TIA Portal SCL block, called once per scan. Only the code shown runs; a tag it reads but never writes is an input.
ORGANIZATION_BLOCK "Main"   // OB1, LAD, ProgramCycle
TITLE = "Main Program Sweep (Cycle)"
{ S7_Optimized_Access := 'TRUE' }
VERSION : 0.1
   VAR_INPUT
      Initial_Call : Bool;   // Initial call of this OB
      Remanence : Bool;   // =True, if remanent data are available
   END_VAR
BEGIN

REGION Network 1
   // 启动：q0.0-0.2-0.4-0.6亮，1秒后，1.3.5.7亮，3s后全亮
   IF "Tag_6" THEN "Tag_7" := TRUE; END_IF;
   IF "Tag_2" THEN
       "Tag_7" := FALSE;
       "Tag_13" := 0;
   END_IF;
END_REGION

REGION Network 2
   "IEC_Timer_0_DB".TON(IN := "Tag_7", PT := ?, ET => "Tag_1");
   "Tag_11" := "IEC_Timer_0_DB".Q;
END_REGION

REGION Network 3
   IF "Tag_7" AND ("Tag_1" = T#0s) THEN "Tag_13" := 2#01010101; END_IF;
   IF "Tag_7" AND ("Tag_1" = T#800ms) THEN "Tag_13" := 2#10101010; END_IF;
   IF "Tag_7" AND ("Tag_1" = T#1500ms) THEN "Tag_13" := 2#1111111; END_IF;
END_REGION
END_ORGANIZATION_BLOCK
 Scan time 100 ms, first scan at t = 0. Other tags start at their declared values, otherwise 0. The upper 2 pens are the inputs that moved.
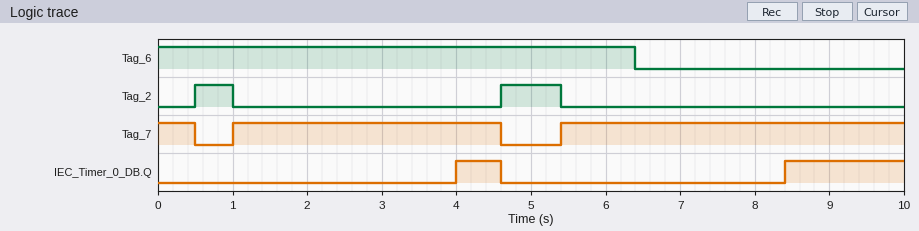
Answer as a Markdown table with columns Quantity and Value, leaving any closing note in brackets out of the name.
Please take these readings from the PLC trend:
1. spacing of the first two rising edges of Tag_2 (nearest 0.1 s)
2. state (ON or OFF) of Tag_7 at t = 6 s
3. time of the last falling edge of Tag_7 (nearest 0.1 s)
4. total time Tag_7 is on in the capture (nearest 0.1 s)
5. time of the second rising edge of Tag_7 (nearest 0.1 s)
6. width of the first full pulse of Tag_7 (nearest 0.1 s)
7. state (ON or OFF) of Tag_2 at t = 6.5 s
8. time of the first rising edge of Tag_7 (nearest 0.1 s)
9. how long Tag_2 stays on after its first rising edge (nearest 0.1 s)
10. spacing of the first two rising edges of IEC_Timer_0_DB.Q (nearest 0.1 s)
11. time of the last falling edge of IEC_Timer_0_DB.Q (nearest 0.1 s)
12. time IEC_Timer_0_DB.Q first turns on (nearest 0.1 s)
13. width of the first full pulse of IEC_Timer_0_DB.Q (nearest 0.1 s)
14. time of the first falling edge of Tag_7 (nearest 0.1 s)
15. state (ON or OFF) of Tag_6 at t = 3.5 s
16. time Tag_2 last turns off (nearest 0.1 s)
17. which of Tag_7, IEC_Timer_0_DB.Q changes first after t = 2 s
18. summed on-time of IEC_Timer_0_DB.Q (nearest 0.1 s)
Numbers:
| Quantity | Value |
|---|---|
| spacing of the first two rising edges of Tag_2 | 4.1 s |
| state (ON or OFF) of Tag_7 at t = 6 s | ON |
| time of the last falling edge of Tag_7 | 4.6 s |
| total time Tag_7 is on in the capture | 8.7 s |
| time of the second rising edge of Tag_7 | 5.4 s |
| width of the first full pulse of Tag_7 | 3.6 s |
| state (ON or OFF) of Tag_2 at t = 6.5 s | OFF |
| time of the first rising edge of Tag_7 | 1.0 s |
| how long Tag_2 stays on after its first rising edge | 0.5 s |
| spacing of the first two rising edges of IEC_Timer_0_DB.Q | 4.4 s |
| time of the last falling edge of IEC_Timer_0_DB.Q | 4.6 s |
| time IEC_Timer_0_DB.Q first turns on | 4.0 s |
| width of the first full pulse of IEC_Timer_0_DB.Q | 0.6 s |
| time of the first falling edge of Tag_7 | 0.5 s |
| state (ON or OFF) of Tag_6 at t = 3.5 s | ON |
| time Tag_2 last turns off | 5.4 s |
| which of Tag_7, IEC_Timer_0_DB.Q changes first after t = 2 s | IEC_Timer_0_DB.Q |
| summed on-time of IEC_Timer_0_DB.Q | 2.2 s |
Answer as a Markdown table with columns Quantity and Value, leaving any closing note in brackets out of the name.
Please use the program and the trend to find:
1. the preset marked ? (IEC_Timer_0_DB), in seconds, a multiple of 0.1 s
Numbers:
| Quantity | Value |
|---|---|
| the preset marked ? (IEC_Timer_0_DB), in seconds, a multiple of 0.1 s | 3.0 s |
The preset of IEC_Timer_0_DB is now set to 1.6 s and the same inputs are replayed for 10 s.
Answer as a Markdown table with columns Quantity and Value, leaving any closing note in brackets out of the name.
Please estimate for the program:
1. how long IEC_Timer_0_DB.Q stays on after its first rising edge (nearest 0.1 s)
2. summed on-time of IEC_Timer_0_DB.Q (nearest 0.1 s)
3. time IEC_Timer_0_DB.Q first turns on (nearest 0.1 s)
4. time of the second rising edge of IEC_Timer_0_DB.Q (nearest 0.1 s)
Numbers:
| Quantity | Value |
|---|---|
| how long IEC_Timer_0_DB.Q stays on after its first rising edge | 2.0 s |
| summed on-time of IEC_Timer_0_DB.Q | 5.0 s |
| time IEC_Timer_0_DB.Q first turns on | 2.6 s |
| time of the second rising edge of IEC_Timer_0_DB.Q | 7.0 s |
